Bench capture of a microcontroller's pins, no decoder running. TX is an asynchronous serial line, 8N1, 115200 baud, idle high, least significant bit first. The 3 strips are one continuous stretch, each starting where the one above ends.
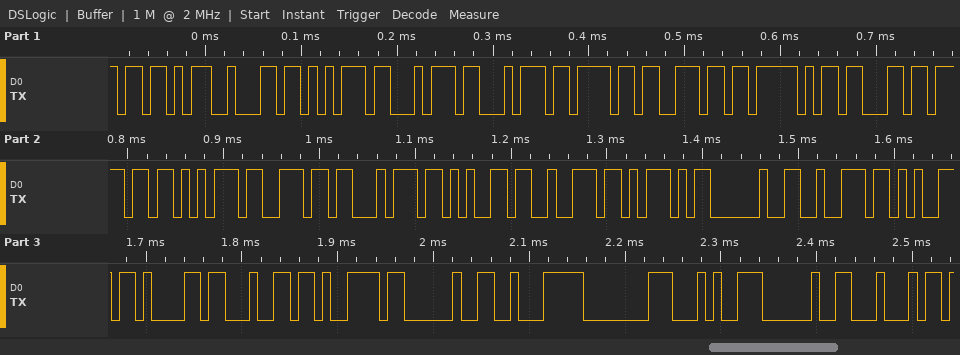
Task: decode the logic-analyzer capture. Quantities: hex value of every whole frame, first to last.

5B 62 75 74 74 6F 6E 5F 63 6F 75 6E 74 65 72 5D 20 72 65 61 64 79 20 E2 80 94 20 44
